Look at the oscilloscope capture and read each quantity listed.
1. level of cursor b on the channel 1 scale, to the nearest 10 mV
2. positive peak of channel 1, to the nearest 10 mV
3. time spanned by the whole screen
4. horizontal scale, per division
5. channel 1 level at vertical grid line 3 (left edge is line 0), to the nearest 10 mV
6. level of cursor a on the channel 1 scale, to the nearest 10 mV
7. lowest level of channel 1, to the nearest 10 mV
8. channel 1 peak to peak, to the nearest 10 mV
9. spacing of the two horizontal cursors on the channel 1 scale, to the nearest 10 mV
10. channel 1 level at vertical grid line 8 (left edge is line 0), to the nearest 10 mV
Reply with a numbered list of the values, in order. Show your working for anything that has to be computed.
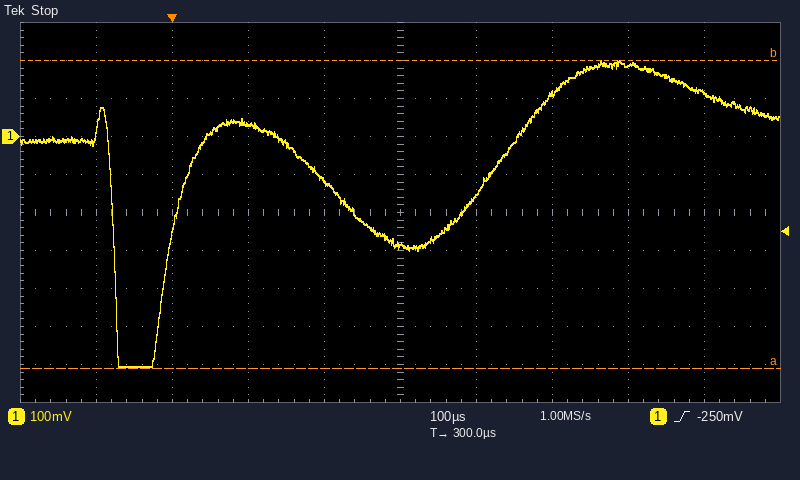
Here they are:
1. 200 mV
2. 200 mV
3. 1 ms
4. 100 µs
5. 30 mV
6. -610 mV
7. -610 mV
8. 200 mV − (-610 mV) = 810 mV
9. 810 mV
10. 190 mV
